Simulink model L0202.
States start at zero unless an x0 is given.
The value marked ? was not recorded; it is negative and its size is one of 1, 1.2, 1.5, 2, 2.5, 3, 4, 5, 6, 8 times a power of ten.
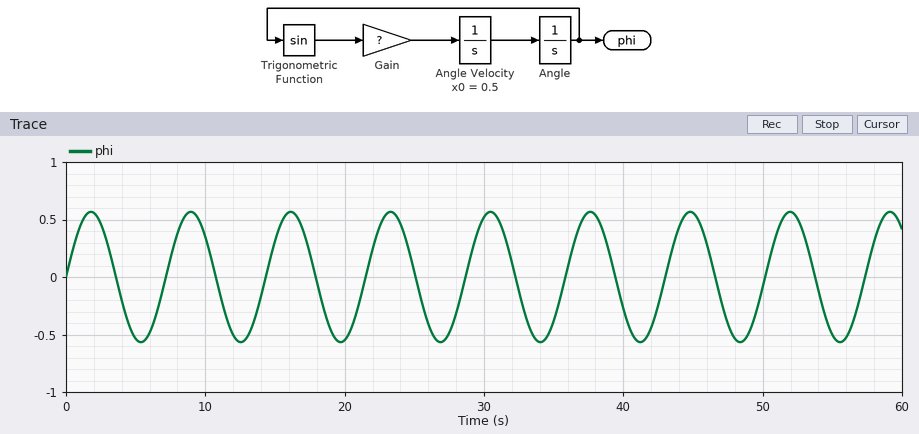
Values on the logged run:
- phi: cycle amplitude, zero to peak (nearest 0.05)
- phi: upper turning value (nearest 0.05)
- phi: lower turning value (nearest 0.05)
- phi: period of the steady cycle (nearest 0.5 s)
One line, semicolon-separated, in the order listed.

0.55; 0.55; -0.55; 7.0 s
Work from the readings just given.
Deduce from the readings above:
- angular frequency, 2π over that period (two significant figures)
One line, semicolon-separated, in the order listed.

0.90 rad/s
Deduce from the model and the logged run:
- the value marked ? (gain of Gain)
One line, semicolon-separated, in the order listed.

-0.8
